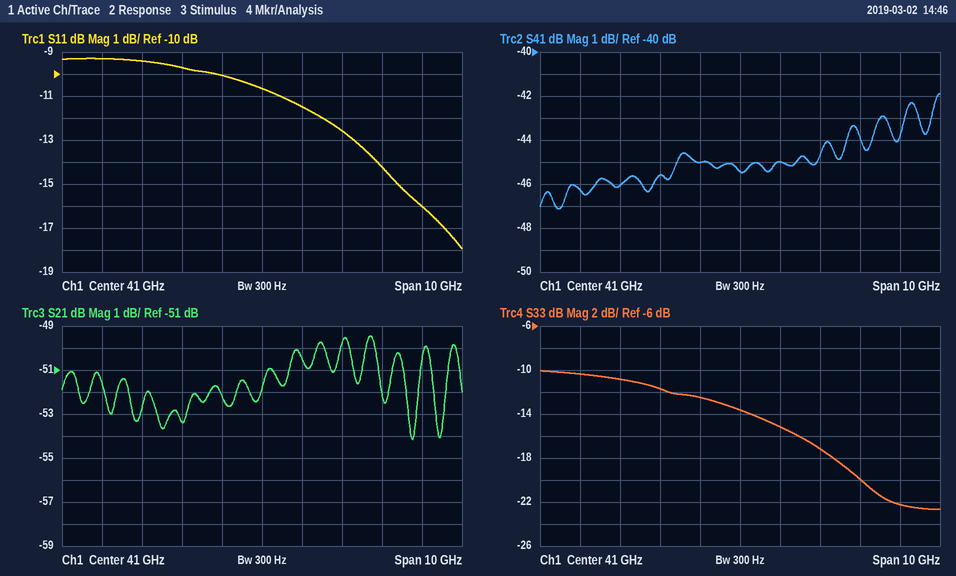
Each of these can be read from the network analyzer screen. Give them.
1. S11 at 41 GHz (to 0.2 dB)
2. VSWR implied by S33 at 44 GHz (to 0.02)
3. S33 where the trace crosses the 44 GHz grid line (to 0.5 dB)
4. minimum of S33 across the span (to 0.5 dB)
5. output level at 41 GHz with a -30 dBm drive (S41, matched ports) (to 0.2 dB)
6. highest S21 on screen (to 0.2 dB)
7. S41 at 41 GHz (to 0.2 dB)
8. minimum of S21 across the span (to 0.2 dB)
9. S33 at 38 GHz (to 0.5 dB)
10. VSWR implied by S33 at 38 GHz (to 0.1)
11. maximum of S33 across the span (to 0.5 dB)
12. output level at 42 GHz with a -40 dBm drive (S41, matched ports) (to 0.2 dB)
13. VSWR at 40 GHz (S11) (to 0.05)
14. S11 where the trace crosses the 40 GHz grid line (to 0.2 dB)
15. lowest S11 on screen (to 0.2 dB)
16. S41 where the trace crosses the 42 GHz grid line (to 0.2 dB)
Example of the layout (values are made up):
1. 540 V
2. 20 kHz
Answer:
1. -10.6 dB
2. 1.22
3. -20.0 dB
4. -22.5 dB
5. -75.4 dBm
6. -49.4 dB
7. -45.4 dB
8. -54.2 dB
9. -11.0 dB
10. 1.8
11. -10.0 dB
12. -85.0 dBm
13. 1.90
14. -10.0 dB
15. -18.0 dB
16. -45.0 dB
